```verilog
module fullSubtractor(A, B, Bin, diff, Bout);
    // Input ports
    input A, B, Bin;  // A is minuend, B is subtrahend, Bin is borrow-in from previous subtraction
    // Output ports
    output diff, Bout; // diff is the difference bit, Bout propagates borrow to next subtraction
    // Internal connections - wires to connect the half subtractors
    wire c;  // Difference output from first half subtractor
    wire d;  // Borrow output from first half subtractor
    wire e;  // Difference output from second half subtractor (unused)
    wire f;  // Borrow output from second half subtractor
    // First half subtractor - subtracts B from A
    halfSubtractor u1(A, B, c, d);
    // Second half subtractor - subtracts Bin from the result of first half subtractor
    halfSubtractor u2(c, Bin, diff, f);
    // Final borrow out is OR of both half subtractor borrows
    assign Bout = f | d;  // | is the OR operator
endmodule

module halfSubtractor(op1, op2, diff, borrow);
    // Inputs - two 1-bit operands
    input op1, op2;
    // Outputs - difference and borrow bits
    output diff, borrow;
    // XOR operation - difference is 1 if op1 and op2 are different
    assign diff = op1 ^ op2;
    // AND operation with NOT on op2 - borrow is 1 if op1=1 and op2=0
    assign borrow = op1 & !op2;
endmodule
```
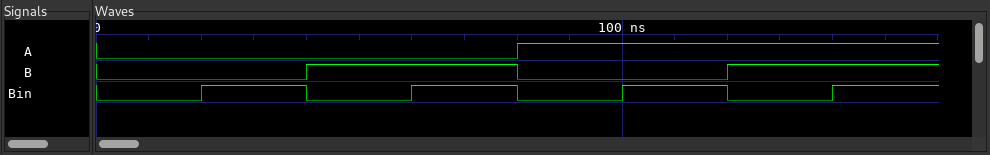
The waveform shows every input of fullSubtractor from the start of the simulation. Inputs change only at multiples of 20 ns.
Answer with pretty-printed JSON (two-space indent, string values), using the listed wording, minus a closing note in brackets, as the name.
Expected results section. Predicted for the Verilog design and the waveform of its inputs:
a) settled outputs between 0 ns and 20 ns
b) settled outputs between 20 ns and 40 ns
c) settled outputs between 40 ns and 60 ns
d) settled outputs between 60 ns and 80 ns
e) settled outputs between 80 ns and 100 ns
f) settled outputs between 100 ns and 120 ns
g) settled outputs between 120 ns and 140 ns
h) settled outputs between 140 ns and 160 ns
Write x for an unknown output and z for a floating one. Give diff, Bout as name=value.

{
  "settled outputs between 0 ns and 20 ns": "diff=0, Bout=0",
  "settled outputs between 20 ns and 40 ns": "diff=1, Bout=0",
  "settled outputs between 40 ns and 60 ns": "diff=1, Bout=1",
  "settled outputs between 60 ns and 80 ns": "diff=0, Bout=0",
  "settled outputs between 80 ns and 100 ns": "diff=1, Bout=1",
  "settled outputs between 100 ns and 120 ns": "diff=0, Bout=1",
  "settled outputs between 120 ns and 140 ns": "diff=0, Bout=0",
  "settled outputs between 140 ns and 160 ns": "diff=1, Bout=0"
}
